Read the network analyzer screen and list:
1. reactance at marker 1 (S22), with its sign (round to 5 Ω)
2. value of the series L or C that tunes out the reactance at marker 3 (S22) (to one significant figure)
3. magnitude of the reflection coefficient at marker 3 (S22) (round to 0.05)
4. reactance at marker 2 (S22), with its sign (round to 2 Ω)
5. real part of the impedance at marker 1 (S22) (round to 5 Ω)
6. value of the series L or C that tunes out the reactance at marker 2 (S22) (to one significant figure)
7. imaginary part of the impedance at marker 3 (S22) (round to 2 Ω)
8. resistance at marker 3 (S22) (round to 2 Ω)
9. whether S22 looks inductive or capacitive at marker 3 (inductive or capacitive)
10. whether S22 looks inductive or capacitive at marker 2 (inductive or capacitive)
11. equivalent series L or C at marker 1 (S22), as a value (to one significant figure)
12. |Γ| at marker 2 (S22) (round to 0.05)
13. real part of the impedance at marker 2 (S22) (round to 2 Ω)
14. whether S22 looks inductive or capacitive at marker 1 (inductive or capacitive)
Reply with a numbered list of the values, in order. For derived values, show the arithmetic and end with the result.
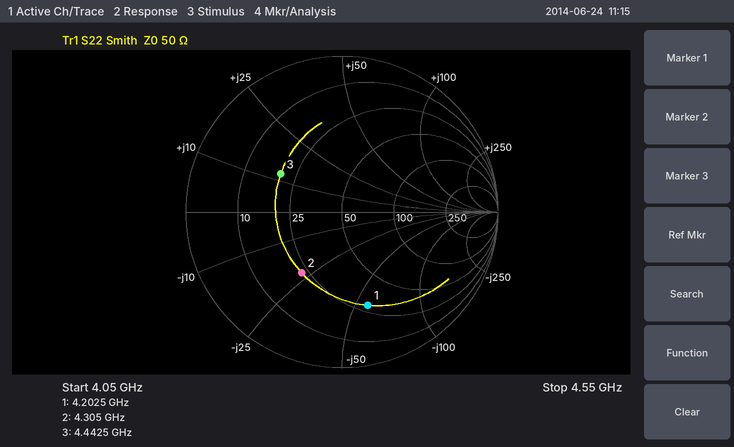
1. -55 Ω
2. C = 1/(2π × 4.4425 GHz × 12 Ω) ≈ 3 pF
3. 0.45
4. -22 Ω
5. 30 Ω
6. L = 22 Ω/(2π × 4.305 GHz) ≈ 813 pH, so 800 pH to one significant figure
7. +12 Ω
8. 20 Ω
9. inductive
10. capacitive
11. C = 1/(2π × 4.2025 GHz × 55 Ω) ≈ 689 fF, so 700 fF to one significant figure
12. 0.45
13. 22 Ω
14. capacitive
